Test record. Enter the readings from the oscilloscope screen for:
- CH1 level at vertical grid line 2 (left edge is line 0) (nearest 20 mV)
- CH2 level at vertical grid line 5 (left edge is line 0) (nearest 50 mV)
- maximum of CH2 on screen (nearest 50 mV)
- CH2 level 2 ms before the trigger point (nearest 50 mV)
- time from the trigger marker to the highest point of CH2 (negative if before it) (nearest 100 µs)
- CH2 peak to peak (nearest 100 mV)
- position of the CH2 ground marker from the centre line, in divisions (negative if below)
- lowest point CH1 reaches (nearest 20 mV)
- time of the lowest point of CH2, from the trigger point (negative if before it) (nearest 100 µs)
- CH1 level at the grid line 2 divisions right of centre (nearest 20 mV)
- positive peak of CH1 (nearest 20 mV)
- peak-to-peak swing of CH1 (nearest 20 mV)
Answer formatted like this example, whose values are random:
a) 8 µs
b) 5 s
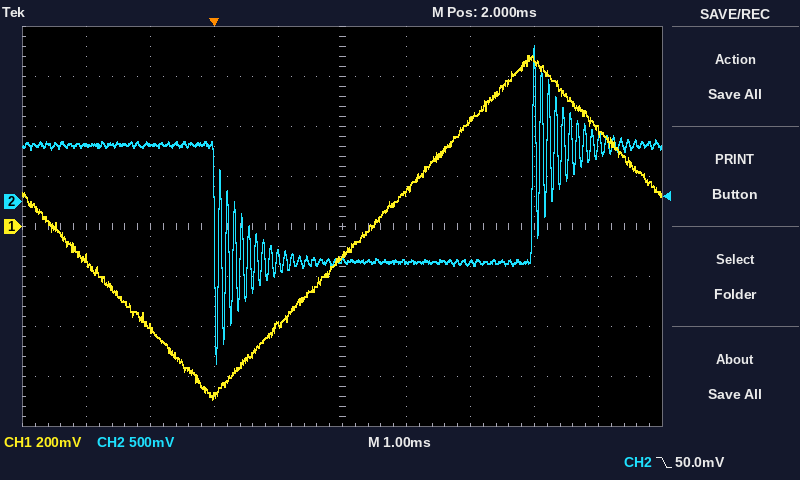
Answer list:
a) -400 mV
b) -600 mV
c) 1.55 V
d) 550 mV
e) +5.0 ms
f) 3.20 V
g) +0.5 div
h) -700 mV
i) 0.0 ms
j) 420 mV
k) 680 mV
l) 1.38 V
